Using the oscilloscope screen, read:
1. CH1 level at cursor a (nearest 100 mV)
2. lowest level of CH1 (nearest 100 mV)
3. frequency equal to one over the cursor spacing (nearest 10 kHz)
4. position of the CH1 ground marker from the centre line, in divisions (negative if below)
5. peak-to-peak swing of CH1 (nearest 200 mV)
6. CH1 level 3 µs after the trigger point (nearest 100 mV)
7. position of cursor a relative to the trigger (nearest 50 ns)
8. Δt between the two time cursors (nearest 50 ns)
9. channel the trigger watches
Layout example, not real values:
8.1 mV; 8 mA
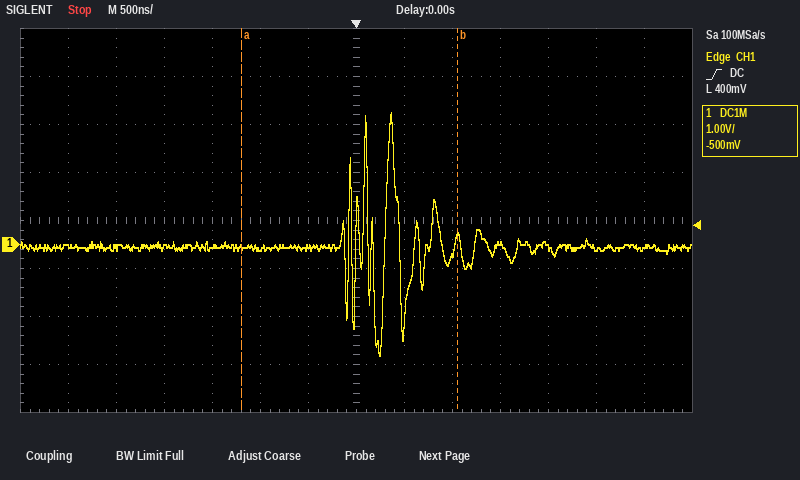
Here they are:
-100 mV; -2.3 V; 440 kHz; -0.5 div; 5.0 V; -100 mV; -1.20 µs; 2.25 µs; CH1
